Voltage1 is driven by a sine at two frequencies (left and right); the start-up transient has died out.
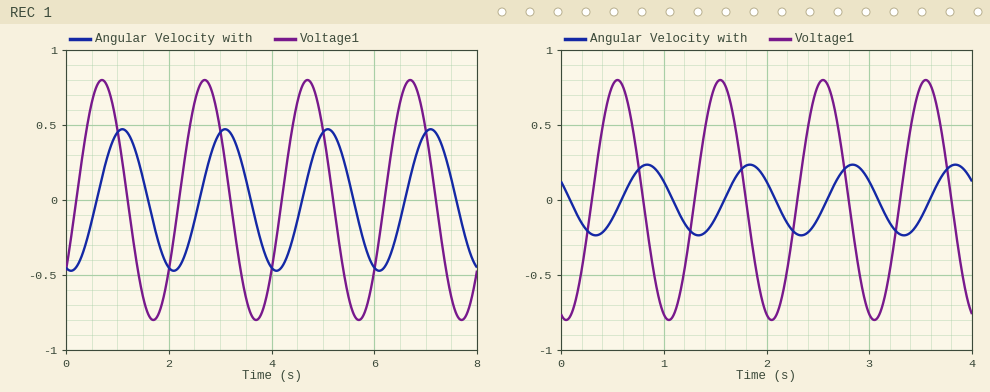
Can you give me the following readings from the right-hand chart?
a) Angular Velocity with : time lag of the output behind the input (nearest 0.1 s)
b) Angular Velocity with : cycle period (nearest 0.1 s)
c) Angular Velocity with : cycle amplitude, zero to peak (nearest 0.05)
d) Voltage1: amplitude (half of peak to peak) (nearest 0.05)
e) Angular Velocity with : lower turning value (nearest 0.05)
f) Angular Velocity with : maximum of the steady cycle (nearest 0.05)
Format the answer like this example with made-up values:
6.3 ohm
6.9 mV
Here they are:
0.3 s
1.0 s
0.25
0.80
-0.25
0.25
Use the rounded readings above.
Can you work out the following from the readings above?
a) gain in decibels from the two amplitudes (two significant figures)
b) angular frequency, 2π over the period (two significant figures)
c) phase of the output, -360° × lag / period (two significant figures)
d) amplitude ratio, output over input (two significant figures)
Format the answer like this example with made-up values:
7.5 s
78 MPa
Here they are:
-10 dB
6.3 rad/s
-110°
0.31
